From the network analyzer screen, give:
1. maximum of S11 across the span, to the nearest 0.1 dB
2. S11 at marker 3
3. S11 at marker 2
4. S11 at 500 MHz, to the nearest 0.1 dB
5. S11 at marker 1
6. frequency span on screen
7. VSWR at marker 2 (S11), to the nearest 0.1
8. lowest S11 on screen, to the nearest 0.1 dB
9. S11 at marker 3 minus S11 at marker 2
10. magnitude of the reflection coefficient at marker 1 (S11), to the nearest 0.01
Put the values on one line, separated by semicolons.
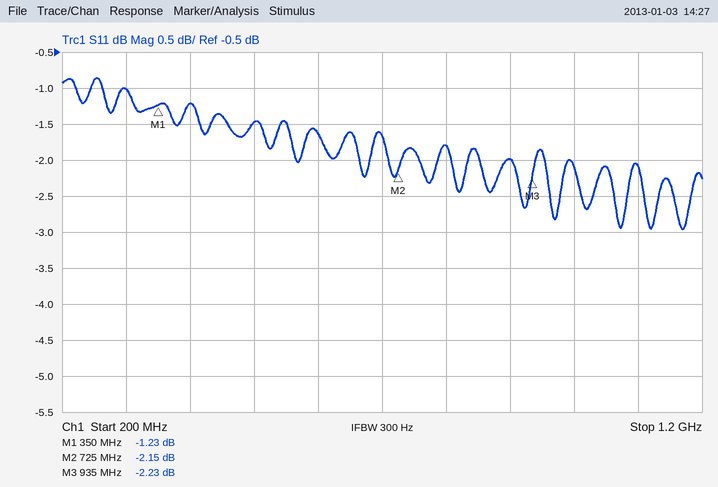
-0.9 dB; -2.23 dB; -2.15 dB; -1.5 dB; -1.23 dB; 1 GHz; 8.1; -3.0 dB; -0.08 dB; 0.87
